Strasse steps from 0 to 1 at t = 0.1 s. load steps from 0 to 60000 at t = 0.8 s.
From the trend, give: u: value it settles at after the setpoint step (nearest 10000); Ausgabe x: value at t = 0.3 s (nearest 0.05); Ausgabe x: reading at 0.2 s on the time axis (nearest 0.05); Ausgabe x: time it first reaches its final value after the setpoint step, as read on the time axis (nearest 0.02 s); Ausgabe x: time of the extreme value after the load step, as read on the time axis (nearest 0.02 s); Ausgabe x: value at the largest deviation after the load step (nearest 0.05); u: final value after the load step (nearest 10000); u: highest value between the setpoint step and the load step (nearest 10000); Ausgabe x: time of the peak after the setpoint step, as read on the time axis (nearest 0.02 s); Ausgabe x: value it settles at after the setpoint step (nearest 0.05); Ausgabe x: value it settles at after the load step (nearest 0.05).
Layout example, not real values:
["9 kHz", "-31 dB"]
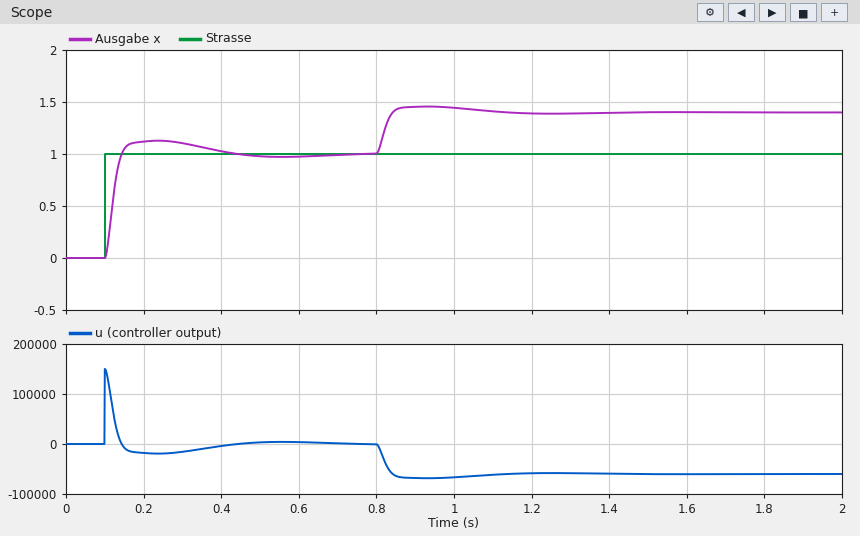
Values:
["0", "1.10", "1.10", "0.14 s", "0.94 s", "1.45", "-60000", "150000", "0.24 s", "1.00", "1.40"]
